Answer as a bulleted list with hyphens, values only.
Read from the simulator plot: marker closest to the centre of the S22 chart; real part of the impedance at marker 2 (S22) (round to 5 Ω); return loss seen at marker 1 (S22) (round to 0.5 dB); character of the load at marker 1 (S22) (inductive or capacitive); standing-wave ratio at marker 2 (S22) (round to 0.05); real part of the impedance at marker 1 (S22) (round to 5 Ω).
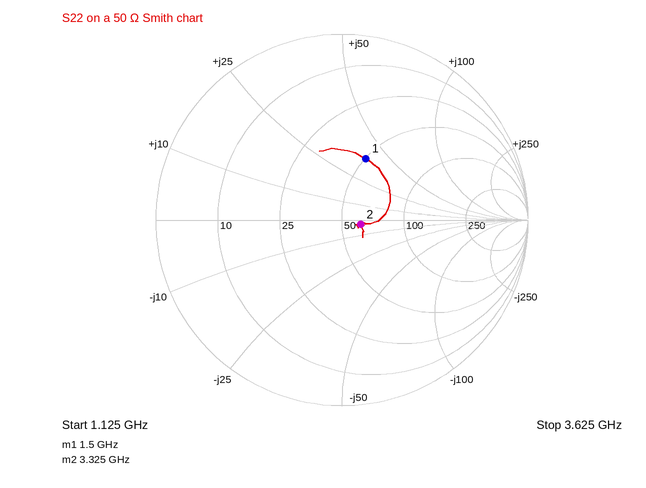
- marker 2
- 60 Ω
- 9.0 dB
- inductive
- 1.25
- 50 Ω
